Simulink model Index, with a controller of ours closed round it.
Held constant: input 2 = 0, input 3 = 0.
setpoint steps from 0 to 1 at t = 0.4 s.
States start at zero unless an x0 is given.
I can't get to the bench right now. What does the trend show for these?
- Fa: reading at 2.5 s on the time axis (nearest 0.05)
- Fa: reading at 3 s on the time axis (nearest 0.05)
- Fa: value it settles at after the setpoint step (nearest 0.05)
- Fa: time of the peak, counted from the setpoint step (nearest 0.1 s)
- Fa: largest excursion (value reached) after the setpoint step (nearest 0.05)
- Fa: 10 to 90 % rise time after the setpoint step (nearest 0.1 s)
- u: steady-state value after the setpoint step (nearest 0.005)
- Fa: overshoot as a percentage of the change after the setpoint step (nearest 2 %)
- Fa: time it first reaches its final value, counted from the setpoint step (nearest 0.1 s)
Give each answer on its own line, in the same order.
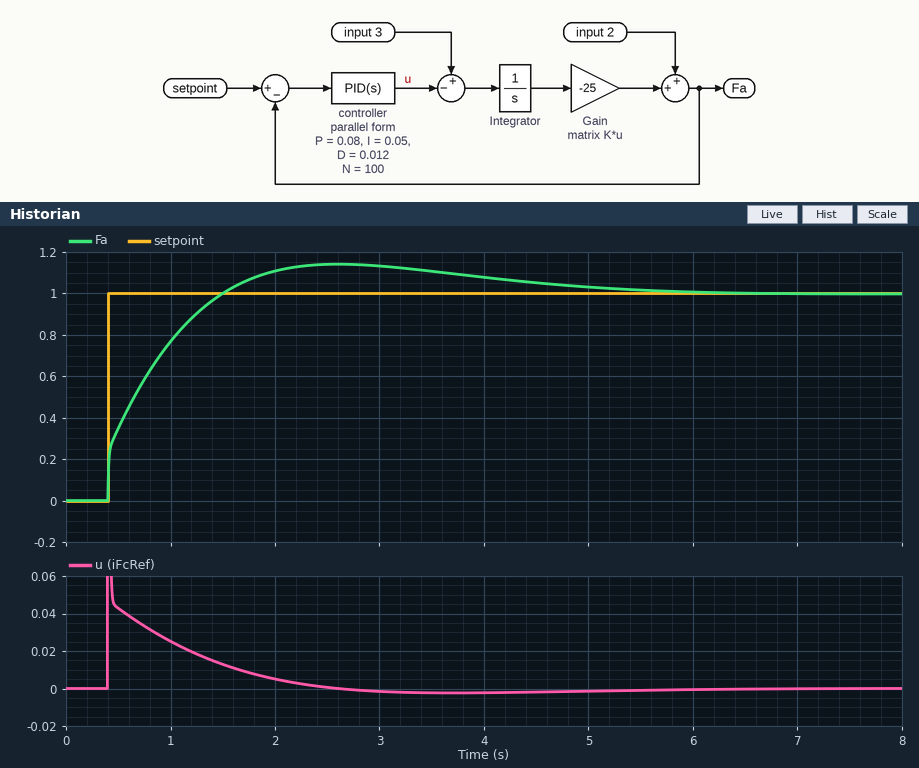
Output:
1.15
1.15
1.00
2.2 s
1.15
0.8 s
0.000
14 %
1.1 s
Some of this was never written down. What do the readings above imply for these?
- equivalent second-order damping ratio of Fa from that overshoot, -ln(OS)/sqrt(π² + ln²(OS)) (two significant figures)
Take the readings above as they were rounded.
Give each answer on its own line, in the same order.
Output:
0.53
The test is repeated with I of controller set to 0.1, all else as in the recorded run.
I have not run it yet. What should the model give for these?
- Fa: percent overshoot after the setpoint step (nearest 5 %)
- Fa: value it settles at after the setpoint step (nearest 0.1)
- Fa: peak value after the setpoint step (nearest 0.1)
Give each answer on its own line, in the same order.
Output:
20 %
1.0
1.2
